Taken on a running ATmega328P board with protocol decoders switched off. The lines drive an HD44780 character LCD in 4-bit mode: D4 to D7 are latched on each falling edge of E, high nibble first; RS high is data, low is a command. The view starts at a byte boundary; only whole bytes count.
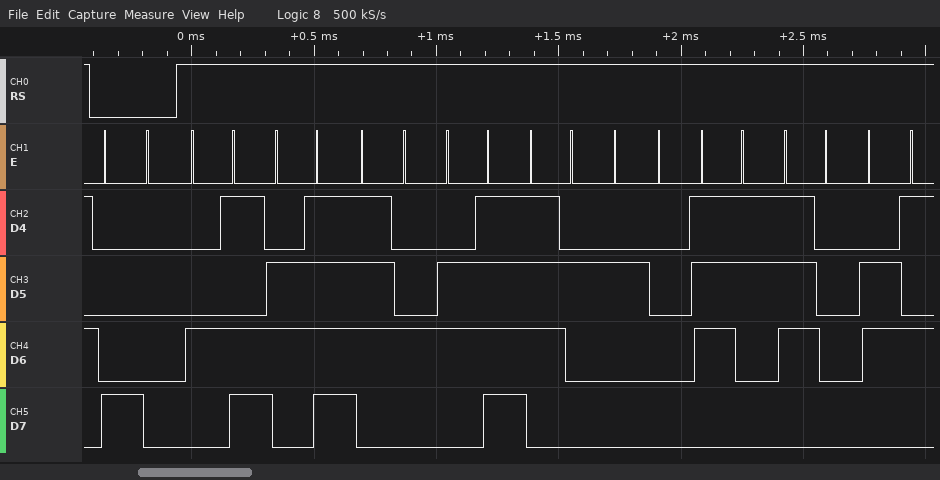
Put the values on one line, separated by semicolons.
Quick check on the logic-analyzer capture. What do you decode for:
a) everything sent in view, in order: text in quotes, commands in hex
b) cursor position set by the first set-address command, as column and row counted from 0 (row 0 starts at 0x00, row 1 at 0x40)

0x80 "Motor spe"; column 0, row 0
